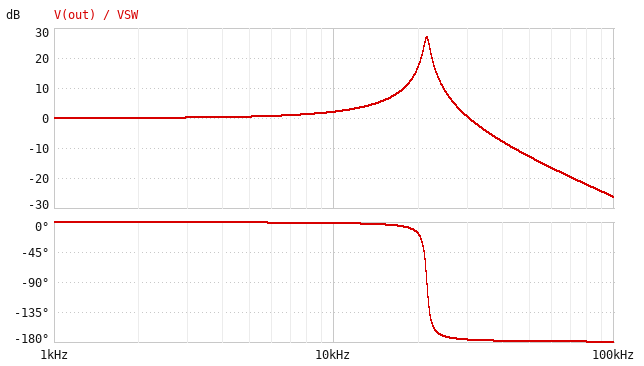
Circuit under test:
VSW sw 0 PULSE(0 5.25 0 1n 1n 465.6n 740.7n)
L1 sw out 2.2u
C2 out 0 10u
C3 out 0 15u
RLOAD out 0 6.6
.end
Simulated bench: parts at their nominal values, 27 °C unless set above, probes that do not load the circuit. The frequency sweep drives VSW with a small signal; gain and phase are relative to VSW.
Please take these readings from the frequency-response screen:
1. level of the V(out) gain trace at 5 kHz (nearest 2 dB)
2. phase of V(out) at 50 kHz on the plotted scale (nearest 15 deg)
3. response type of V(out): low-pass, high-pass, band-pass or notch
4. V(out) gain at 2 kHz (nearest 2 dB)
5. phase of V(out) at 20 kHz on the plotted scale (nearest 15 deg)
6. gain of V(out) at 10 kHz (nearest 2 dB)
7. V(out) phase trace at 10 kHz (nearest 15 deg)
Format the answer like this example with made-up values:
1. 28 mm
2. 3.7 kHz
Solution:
1. 0 dB
2. -180 deg
3. low-pass
4. 0 dB
5. -15 deg
6. 2 dB
7. 0 deg
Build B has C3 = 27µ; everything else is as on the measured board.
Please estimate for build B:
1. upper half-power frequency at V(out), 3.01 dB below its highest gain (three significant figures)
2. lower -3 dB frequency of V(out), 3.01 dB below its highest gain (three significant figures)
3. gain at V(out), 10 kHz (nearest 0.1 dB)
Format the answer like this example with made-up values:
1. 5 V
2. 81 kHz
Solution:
1. 18.0 kHz
2. 17.3 kHz
3. 3.4 dB
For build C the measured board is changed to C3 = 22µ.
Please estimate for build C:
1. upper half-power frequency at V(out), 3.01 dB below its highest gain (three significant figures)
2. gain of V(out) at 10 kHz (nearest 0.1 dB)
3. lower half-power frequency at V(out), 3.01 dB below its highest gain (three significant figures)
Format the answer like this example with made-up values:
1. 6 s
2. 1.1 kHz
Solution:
1. 19.3 kHz
2. 2.8 dB
3. 18.6 kHz
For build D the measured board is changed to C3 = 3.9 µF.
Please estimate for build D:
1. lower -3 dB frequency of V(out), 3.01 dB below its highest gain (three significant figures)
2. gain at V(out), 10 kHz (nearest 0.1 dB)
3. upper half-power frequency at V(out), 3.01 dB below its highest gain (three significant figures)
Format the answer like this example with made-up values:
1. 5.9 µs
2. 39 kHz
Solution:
1. 27.9 kHz
2. 1.1 dB
3. 29.6 kHz
